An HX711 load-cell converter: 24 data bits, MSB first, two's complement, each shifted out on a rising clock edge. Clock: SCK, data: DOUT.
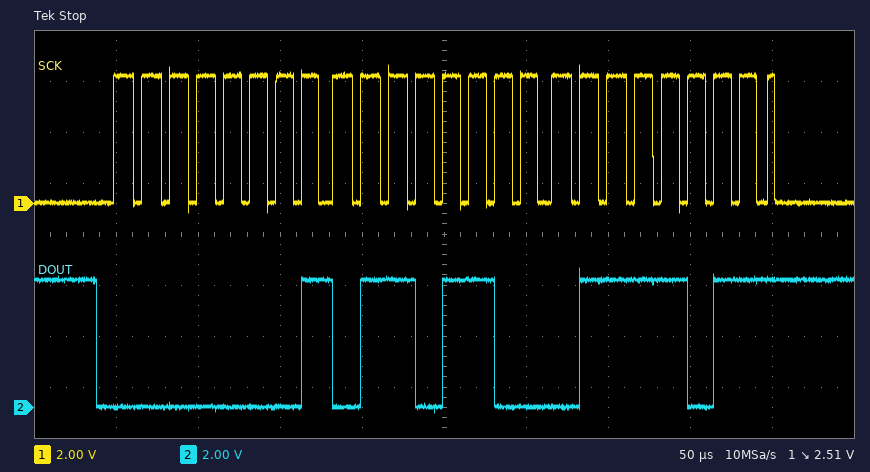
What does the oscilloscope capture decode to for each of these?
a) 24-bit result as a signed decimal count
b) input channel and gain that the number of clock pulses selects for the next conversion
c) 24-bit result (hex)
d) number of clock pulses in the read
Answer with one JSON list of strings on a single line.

["93307", "channel A, gain 128", "0x016C7B", "25"]
